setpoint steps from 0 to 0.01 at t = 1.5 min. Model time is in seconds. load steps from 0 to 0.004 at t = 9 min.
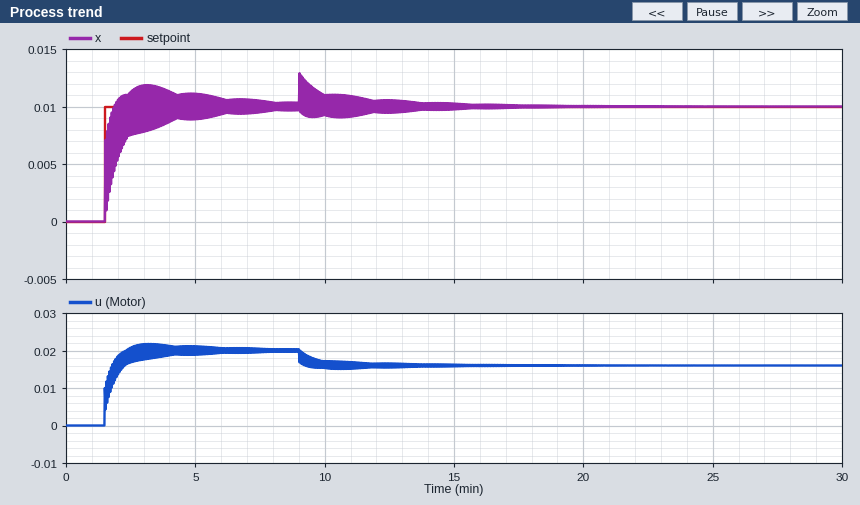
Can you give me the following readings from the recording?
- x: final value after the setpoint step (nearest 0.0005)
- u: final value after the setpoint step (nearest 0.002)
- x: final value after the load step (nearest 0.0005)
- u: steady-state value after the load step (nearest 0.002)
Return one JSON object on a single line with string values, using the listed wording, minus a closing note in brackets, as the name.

{"x: final value after the setpoint step": "0.0100", "u: final value after the setpoint step": "0.020", "x: final value after the load step": "0.0100", "u: steady-state value after the load step": "0.016"}
